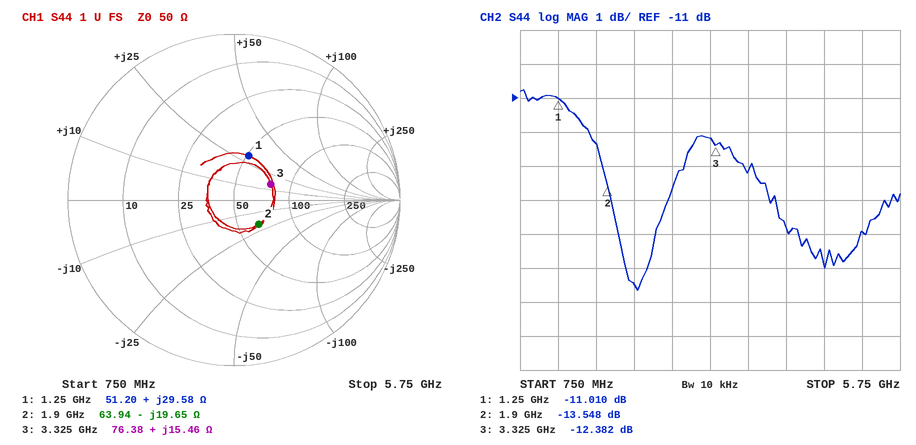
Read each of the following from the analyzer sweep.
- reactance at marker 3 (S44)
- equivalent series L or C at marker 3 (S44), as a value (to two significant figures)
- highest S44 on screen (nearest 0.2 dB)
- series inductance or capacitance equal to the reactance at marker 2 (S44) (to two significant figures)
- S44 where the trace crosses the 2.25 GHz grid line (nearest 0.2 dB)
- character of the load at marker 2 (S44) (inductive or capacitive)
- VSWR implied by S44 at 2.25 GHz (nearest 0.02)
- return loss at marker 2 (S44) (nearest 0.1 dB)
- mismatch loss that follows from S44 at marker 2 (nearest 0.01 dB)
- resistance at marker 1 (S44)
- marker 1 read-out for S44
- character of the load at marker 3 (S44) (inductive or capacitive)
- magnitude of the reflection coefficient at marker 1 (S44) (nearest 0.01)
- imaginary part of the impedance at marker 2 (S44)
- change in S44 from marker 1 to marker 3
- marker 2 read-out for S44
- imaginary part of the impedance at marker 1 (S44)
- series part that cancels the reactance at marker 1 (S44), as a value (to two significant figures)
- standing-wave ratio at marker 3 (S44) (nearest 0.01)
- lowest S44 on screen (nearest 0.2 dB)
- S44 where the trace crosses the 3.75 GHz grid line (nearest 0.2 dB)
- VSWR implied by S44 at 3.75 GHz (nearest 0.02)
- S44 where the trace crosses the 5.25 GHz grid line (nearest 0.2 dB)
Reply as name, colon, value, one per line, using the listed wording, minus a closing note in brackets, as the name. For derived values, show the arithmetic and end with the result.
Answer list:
reactance at marker 3: +15.46 Ω
equivalent series L or C at marker 3 (S44), as a value: L = 15.46 Ω/(2π × 3.325 GHz) ≈ 740 pH
highest S44 on screen: -10.8 dB
series inductance or capacitance equal to the reactance at marker 2 (S44): C = 1/(2π × 1.9 GHz × 19.65 Ω) ≈ 4.3 pF
S44 where the trace crosses the 2.25 GHz grid line: -16.4 dB
character of the load at marker 2 (S44): capacitive
VSWR implied by S44 at 2.25 GHz: |Γ| = 10^(-16.4/20) = 0.1514; VSWR = (1 + 0.1514)/(1 − 0.1514) ≈ 1.36
return loss at marker 2 (S44): 13.6 dB
mismatch loss that follows from S44 at marker 2: −10 log10(1 − 10^(-13.548/10)) ≈ 0.20 dB
resistance at marker 1: 51.20 Ω
marker 1 read-out for S44: -11.010 dB
character of the load at marker 3 (S44): inductive
magnitude of the reflection coefficient at marker 1 (S44): 0.28
imaginary part of the impedance at marker 2: -19.65 Ω
change in S44 from marker 1 to marker 3: -12.382 − (-11.01) = -1.372 dB
marker 2 read-out for S44: -13.548 dB
imaginary part of the impedance at marker 1: +29.58 Ω
series part that cancels the reactance at marker 1 (S44), as a value: C = 1/(2π × 1.25 GHz × 29.58 Ω) ≈ 4.3 pF
standing-wave ratio at marker 3 (S44): 1.63
lowest S44 on screen: -16.6 dB
S44 where the trace crosses the 3.75 GHz grid line: -13.2 dB
VSWR implied by S44 at 3.75 GHz: |Γ| = 10^(-13.2/20) = 0.2188; VSWR = (1 + 0.2188)/(1 − 0.2188) ≈ 1.56
S44 where the trace crosses the 5.25 GHz grid line: -15.0 dB
